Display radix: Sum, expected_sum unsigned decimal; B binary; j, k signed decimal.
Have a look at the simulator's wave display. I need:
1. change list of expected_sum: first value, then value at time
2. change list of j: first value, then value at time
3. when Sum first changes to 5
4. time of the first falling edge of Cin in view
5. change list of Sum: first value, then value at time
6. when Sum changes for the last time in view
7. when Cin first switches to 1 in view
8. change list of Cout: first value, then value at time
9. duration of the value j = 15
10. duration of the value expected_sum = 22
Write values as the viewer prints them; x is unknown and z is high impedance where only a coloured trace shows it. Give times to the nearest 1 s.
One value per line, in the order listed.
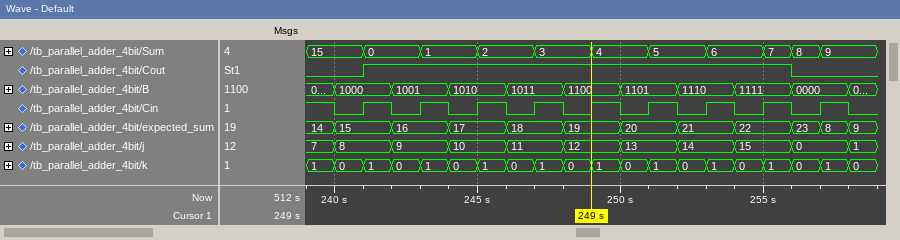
14, 15 at 240 s, 16 at 242 s, 17 at 244 s, 18 at 246 s, 19 at 248 s, 20 at 250 s, 21 at 252 s, 22 at 254 s, 23 at 256 s, 8 at 257 s, 9 at 258 s
7, 8 at 240 s, 9 at 242 s, 10 at 244 s, 11 at 246 s, 12 at 248 s, 13 at 250 s, 14 at 252 s, 15 at 254 s, 0 at 256 s, 1 at 258 s
251 s
240 s
15, 0 at 241 s, 1 at 243 s, 2 at 245 s, 3 at 247 s, 4 at 249 s, 5 at 251 s, 6 at 253 s, 7 at 255 s, 8 at 256 s, 9 at 257 s
257 s
241 s
0, 1 at 241 s, 0 at 256 s
2 s
2 s
